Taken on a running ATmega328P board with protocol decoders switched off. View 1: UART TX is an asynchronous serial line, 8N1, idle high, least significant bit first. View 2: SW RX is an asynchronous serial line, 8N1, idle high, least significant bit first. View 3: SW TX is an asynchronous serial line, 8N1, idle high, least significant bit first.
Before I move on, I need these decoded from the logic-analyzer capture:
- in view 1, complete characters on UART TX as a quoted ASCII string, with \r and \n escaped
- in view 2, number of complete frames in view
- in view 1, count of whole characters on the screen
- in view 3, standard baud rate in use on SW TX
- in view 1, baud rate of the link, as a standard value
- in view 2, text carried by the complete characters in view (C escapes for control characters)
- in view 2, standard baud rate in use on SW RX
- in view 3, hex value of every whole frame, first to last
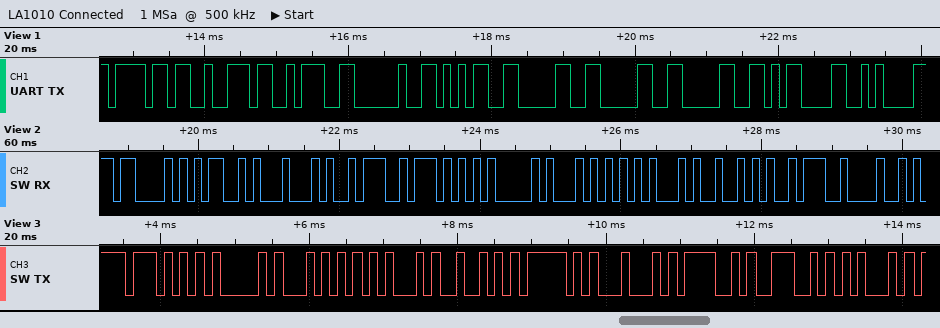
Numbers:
"or: 5000\r\n"
11
10
9600 baud
9600 baud
"CMD:WATER:H"
9600 baud
57 41 54 45 52 5F 44 4F 4E 45
